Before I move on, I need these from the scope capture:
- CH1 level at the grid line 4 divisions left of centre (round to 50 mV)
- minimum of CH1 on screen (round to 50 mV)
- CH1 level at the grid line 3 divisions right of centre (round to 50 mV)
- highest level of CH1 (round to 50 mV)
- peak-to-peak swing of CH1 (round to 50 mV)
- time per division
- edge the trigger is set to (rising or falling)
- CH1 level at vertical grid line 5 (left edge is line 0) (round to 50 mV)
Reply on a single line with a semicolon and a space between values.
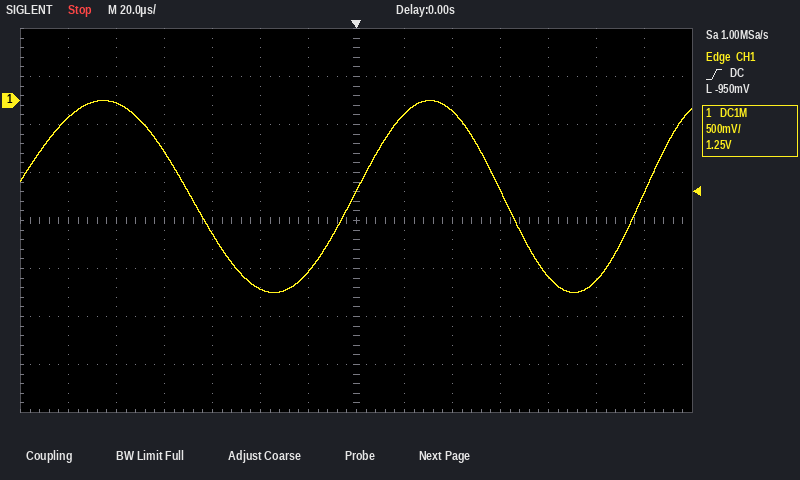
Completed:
-550 mV; -2.00 V; -950 mV; 0 mV; 2.00 V; 20 µs; rising; -1.95 V
